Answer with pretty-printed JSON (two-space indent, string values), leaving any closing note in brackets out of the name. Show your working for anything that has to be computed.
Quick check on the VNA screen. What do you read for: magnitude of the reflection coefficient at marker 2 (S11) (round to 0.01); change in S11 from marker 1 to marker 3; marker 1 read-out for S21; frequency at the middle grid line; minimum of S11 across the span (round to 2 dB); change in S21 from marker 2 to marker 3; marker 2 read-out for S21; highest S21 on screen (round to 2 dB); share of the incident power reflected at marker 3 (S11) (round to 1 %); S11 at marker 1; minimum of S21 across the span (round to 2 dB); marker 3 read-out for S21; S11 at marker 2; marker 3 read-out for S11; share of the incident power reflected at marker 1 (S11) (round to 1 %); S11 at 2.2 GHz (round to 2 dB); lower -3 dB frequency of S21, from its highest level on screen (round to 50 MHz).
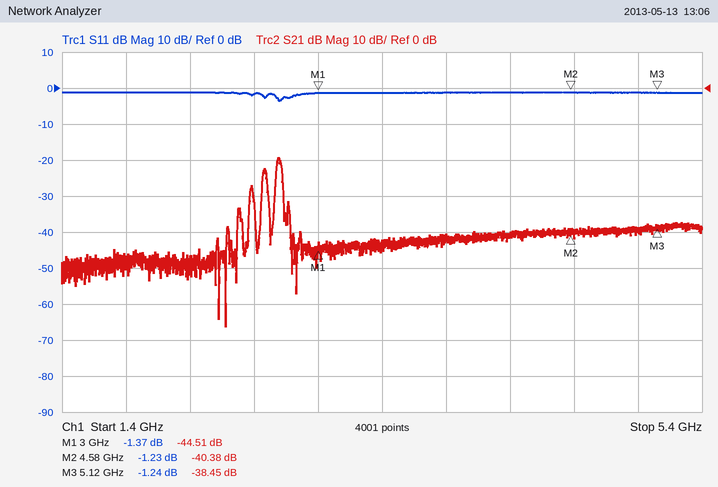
{
  "magnitude of the reflection coefficient at marker 2 (S11)": "10^(-1.23/20) ≈ 0.87",
  "change in S11 from marker 1 to marker 3": "-1.24 − (-1.37) = 0.13 dB",
  "marker 1 read-out for S21": "-44.51 dB",
  "frequency at the middle grid line": "3.4 GHz",
  "minimum of S11 across the span": "-4 dB",
  "change in S21 from marker 2 to marker 3": "-38.45 − (-40.38) = 1.93 dB",
  "marker 2 read-out for S21": "-40.38 dB",
  "highest S21 on screen": "-20 dB",
  "share of the incident power reflected at marker 3 (S11)": "10^(-1.24/10) ≈ 75 %",
  "S11 at marker 1": "-1.37 dB",
  "minimum of S21 across the span": "-66 dB",
  "marker 3 read-out for S21": "-38.45 dB",
  "S11 at marker 2": "-1.23 dB",
  "marker 3 read-out for S11": "-1.24 dB",
  "share of the incident power reflected at marker 1 (S11)": "10^(-1.37/10) ≈ 73 %",
  "S11 at 2.2 GHz": "-2 dB",
  "lower -3 dB frequency of S21, from its highest level on screen": "2.75 GHz"
}
